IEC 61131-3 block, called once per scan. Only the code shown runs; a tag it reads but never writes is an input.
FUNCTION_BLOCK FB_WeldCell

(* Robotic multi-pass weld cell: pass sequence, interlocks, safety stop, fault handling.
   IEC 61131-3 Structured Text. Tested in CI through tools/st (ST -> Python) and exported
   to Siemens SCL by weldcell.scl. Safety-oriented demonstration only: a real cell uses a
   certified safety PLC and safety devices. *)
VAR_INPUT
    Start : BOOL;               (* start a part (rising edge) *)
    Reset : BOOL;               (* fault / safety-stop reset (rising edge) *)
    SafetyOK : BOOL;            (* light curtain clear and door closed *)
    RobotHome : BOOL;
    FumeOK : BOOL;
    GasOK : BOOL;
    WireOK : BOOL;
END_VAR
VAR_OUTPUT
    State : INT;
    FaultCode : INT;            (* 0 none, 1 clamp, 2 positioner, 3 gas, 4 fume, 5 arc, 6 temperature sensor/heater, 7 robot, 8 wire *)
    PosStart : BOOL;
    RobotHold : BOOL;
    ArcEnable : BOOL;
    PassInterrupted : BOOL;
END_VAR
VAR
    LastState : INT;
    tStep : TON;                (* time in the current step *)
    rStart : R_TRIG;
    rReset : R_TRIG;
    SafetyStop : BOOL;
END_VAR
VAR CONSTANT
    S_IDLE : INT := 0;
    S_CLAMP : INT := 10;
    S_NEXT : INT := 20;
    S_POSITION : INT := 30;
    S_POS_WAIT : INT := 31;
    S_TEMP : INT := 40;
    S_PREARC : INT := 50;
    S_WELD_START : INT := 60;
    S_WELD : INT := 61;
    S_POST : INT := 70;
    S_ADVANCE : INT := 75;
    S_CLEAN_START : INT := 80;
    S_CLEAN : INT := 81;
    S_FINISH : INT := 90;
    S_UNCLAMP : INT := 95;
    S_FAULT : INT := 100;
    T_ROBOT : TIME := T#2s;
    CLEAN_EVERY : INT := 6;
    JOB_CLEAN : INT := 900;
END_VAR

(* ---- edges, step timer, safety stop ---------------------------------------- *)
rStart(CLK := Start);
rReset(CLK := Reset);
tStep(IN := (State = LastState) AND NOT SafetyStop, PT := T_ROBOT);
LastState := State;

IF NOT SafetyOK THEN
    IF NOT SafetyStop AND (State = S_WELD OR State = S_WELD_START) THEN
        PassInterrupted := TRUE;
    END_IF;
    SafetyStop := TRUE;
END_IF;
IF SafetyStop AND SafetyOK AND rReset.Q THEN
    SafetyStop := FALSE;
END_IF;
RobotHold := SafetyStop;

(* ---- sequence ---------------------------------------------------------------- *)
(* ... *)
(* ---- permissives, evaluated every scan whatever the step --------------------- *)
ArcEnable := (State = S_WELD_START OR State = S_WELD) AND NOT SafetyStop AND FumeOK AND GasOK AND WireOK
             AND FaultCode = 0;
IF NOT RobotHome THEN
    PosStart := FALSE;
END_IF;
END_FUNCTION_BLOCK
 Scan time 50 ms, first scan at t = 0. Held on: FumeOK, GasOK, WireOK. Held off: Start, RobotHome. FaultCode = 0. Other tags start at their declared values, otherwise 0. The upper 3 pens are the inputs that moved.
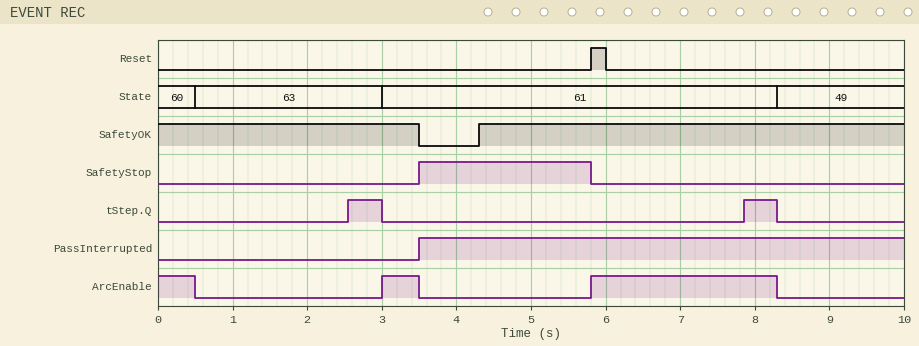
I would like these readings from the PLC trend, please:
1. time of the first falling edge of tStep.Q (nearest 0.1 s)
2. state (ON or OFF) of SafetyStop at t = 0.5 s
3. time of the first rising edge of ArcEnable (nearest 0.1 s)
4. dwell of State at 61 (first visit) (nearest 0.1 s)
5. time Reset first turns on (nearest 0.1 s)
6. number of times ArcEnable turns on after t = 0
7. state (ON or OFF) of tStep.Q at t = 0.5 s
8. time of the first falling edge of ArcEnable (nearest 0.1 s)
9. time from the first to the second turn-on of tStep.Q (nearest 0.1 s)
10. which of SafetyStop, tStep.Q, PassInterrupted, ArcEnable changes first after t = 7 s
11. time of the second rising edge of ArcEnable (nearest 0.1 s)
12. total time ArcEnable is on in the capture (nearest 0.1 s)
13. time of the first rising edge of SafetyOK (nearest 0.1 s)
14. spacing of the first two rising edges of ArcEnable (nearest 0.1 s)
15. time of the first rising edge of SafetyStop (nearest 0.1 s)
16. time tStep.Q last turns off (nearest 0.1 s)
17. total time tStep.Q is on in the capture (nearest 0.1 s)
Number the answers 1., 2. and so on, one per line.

1. 3.0 s
2. OFF
3. 3.0 s
4. 5.3 s
5. 5.8 s
6. 2
7. OFF
8. 0.5 s
9. 5.3 s
10. tStep.Q
11. 5.8 s
12. 3.5 s
13. 4.3 s
14. 2.8 s
15. 3.5 s
16. 8.3 s
17. 0.9 s
